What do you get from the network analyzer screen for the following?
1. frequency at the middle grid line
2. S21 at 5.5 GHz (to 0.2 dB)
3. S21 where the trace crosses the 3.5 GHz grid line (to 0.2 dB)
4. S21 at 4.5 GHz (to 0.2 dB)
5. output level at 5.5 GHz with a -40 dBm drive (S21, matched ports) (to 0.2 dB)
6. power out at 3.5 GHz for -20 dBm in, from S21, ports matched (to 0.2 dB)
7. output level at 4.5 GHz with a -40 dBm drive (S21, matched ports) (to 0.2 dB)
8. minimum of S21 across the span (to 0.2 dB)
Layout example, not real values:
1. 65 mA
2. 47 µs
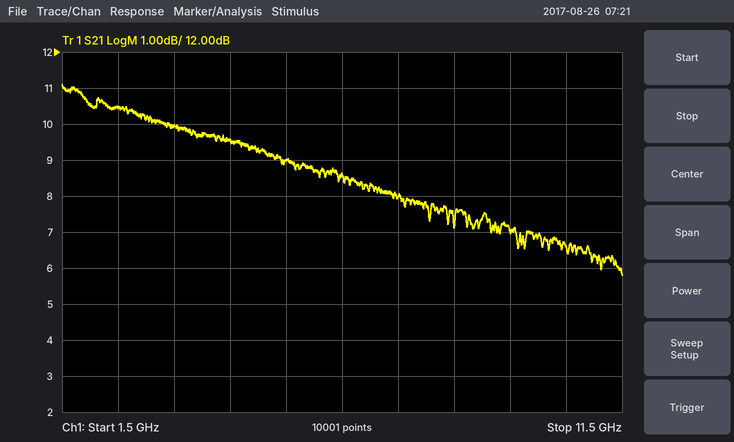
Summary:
1. 6.5 GHz
2. 9.0 dB
3. 10.0 dB
4. 9.6 dB
5. -31.0 dBm
6. -10.0 dBm
7. -30.4 dBm
8. 5.8 dB
